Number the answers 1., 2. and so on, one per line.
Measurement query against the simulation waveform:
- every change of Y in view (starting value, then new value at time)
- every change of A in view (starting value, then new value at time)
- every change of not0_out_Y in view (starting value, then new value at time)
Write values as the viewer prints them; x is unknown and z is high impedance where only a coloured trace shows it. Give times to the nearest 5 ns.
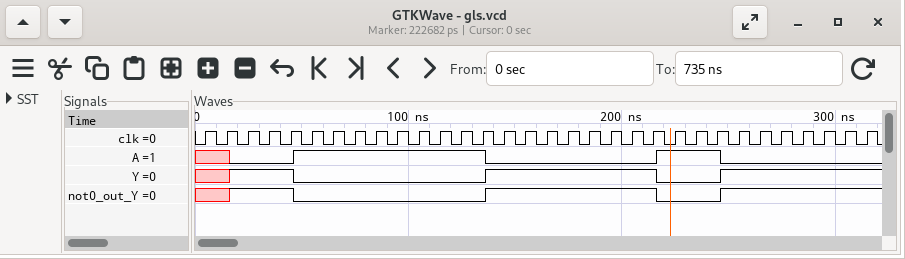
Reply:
1. x, 1 at 15 ns, 0 at 45 ns, 1 at 135 ns, 0 at 215 ns, 1 at 245 ns
2. x, 0 at 15 ns, 1 at 45 ns, 0 at 135 ns, 1 at 215 ns, 0 at 245 ns
3. x, 1 at 15 ns, 0 at 45 ns, 1 at 135 ns, 0 at 215 ns, 1 at 245 ns
